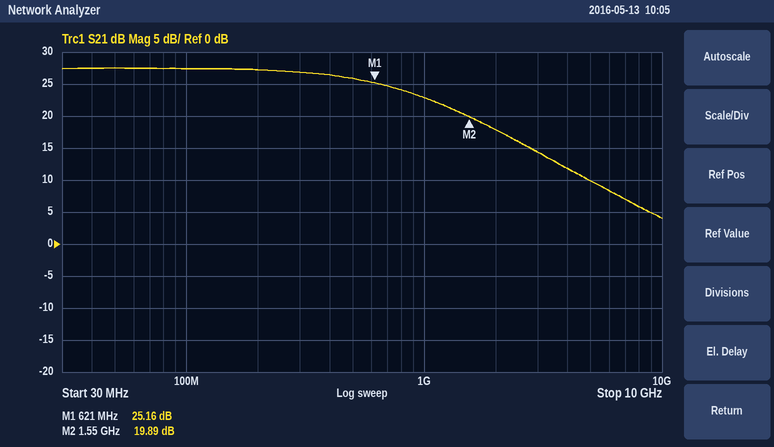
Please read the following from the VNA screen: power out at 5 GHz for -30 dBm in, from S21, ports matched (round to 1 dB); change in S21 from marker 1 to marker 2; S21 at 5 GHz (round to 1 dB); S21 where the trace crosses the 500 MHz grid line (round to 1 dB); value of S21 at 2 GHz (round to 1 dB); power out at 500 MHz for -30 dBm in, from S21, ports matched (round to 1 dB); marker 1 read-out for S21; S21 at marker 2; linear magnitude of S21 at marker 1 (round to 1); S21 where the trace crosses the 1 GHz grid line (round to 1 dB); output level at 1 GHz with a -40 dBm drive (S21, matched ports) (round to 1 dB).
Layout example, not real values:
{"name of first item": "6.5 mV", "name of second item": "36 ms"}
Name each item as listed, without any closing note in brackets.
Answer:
{"power out at 5 GHz for -30 dBm in, from S21, ports matched": "-20 dBm", "change in S21 from marker 1 to marker 2": "-5.27 dB", "S21 at 5 GHz": "10 dB", "S21 where the trace crosses the 500 MHz grid line": "26 dB", "value of S21 at 2 GHz": "18 dB", "power out at 500 MHz for -30 dBm in, from S21, ports matched": "-4 dBm", "marker 1 read-out for S21": "25.16 dB", "S21 at marker 2": "19.89 dB", "linear magnitude of S21 at marker 1": "18", "S21 where the trace crosses the 1 GHz grid line": "23 dB", "output level at 1 GHz with a -40 dBm drive (S21, matched ports)": "-17 dBm"}
